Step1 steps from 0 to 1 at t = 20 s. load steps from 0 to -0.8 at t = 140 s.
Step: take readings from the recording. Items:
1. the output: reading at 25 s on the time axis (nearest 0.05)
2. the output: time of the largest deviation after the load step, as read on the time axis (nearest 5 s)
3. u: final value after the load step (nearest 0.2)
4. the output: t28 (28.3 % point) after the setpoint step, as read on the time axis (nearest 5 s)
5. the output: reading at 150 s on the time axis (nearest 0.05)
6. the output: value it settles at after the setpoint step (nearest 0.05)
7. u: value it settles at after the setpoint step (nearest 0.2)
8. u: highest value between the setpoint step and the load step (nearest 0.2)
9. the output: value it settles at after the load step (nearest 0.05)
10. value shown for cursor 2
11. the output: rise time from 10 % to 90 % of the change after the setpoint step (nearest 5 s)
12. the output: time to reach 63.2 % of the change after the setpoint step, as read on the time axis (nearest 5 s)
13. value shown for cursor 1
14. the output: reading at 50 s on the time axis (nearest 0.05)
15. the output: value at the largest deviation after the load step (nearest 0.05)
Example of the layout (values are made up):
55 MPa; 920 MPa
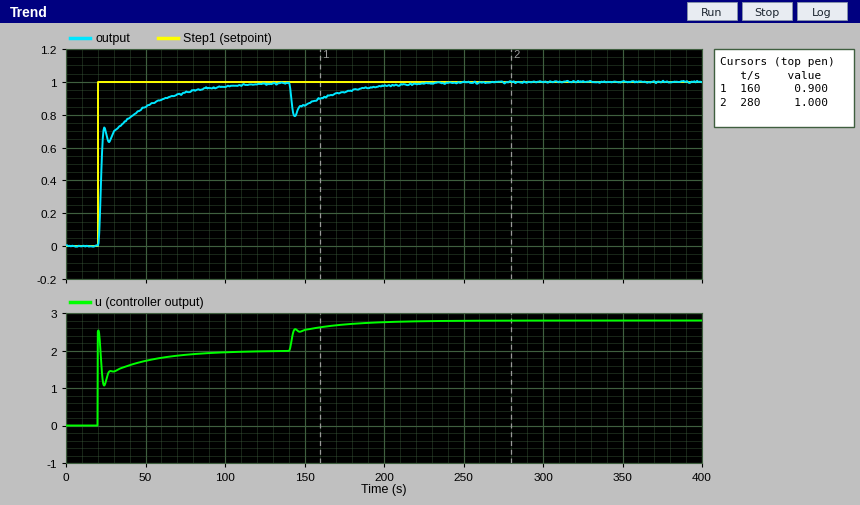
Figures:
0.70; 145 s; 2.8; 20 s; 0.85; 1.00; 2.0; 2.6; 1.00; 1.000; 40 s; 25 s; 0.900; 0.85; 0.80
